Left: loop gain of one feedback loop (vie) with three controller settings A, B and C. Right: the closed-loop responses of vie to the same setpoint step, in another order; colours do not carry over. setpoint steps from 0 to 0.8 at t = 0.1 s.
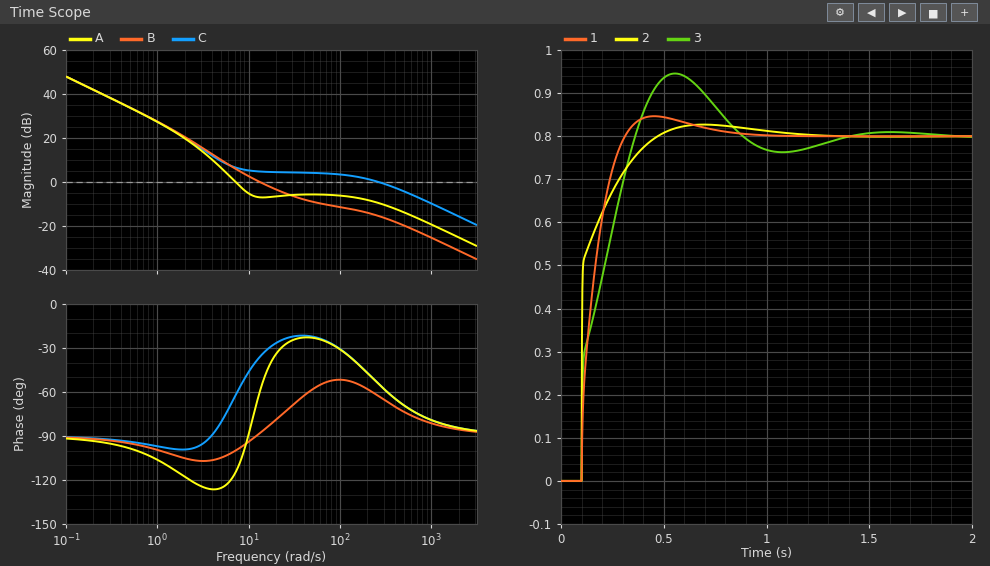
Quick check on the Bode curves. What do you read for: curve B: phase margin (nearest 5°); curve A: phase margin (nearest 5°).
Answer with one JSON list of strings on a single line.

["90°", "65°"]
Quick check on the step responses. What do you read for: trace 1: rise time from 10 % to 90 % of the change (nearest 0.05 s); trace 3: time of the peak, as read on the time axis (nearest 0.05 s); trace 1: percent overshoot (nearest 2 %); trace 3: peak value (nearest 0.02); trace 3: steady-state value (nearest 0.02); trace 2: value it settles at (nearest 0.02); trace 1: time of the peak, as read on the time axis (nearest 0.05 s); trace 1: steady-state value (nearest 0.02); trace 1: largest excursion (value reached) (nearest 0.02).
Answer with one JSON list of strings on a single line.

["0.15 s", "0.55 s", "6 %", "0.94", "0.80", "0.80", "0.45 s", "0.80", "0.84"]
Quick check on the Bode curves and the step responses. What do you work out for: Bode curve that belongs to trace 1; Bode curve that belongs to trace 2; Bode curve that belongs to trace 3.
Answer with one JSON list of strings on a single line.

["B", "C", "A"]
